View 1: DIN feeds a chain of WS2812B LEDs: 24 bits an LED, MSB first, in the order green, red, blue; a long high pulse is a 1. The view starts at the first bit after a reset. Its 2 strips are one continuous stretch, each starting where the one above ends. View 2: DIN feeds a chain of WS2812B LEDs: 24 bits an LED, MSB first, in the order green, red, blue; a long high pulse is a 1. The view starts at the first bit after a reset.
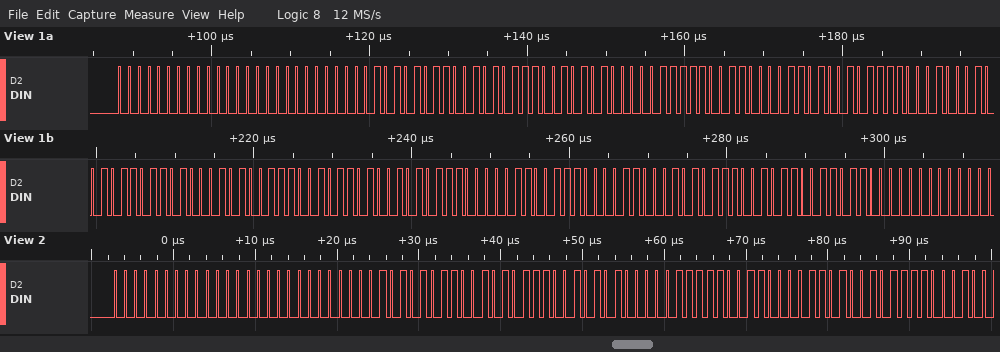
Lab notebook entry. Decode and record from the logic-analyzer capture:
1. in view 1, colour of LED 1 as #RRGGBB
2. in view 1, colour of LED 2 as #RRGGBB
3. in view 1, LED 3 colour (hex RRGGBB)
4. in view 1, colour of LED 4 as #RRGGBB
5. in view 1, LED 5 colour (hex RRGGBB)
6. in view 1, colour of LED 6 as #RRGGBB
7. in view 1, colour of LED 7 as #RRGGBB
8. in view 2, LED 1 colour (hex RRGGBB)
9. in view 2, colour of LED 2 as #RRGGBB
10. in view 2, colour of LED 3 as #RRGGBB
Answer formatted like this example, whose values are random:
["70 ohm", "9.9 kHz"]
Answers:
["#000000", "#CA2AE5", "#F3410D", "#112F2D", "#9CA2B4", "#0CAEE1", "#E58A9B", "#000000", "#CA2AE5", "#F3410D"]
